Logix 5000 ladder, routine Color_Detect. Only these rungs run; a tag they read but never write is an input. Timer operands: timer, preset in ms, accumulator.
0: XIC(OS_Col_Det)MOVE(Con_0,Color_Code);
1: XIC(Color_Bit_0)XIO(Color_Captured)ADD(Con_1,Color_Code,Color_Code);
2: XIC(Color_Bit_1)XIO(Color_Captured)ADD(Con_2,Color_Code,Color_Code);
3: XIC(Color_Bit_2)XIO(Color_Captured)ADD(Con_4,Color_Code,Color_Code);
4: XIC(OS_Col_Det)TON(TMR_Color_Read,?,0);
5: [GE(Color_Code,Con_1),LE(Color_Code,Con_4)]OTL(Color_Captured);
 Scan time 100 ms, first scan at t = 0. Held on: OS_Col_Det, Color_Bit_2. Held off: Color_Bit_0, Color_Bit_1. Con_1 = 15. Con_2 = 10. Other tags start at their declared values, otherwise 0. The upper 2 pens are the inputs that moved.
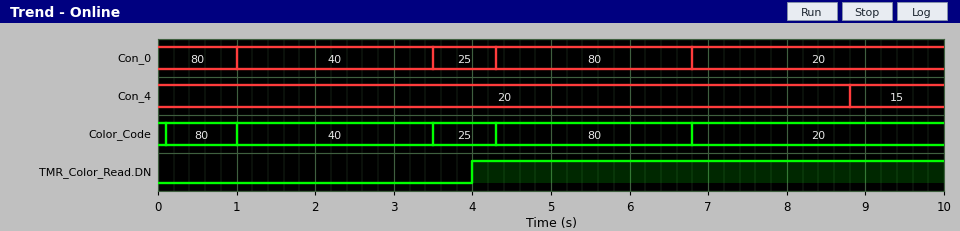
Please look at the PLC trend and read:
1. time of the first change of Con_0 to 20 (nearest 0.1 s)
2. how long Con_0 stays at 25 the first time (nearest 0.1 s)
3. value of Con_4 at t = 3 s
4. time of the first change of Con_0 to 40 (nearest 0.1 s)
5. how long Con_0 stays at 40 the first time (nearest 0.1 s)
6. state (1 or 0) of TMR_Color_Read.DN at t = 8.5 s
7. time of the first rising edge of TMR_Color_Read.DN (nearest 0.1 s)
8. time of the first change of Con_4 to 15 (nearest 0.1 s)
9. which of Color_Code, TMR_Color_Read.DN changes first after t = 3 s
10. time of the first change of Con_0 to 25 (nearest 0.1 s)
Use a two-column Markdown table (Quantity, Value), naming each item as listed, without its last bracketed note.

| Quantity | Value |
|---|---|
| time of the first change of Con_0 to 20 | 6.8 s |
| how long Con_0 stays at 25 the first time | 0.8 s |
| value of Con_4 at t = 3 s | 20 |
| time of the first change of Con_0 to 40 | 1.0 s |
| how long Con_0 stays at 40 the first time | 2.5 s |
| state (1 or 0) of TMR_Color_Read.DN at t = 8.5 s | 1 |
| time of the first rising edge of TMR_Color_Read.DN | 4.0 s |
| time of the first change of Con_4 to 15 | 8.8 s |
| which of Color_Code, TMR_Color_Read.DN changes first after t = 3 s | Color_Code |
| time of the first change of Con_0 to 25 | 3.5 s |
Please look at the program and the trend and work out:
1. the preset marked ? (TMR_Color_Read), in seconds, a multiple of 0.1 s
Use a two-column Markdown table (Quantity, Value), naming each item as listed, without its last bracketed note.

| Quantity | Value |
|---|---|
| the preset marked ? (TMR_Color_Read), in seconds, a multiple of 0.1 s | 4.0 s |
